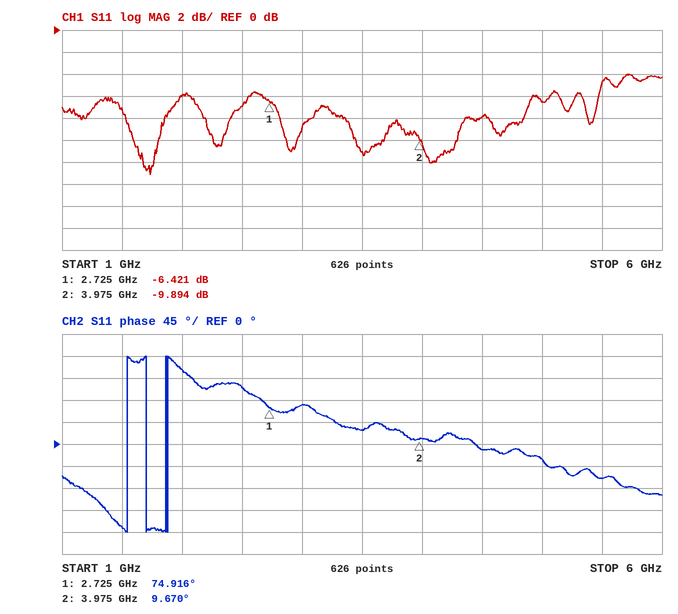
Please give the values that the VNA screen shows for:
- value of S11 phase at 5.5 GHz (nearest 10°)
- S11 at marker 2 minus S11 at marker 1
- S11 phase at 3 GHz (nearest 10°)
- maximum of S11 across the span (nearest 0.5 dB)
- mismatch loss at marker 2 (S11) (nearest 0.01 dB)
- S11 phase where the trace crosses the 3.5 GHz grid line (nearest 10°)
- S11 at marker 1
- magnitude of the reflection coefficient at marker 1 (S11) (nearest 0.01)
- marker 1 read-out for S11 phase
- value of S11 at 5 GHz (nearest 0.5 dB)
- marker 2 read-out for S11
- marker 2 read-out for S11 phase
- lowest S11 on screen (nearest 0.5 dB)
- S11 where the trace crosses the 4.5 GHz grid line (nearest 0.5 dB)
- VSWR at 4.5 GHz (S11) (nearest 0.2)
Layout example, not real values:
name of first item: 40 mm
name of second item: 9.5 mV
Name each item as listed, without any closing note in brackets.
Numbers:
value of S11 phase at 5.5 GHz: -70°
S11 at marker 2 minus S11 at marker 1: -3.473 dB
S11 phase at 3 GHz: 80°
maximum of S11 across the span: -4.0 dB
mismatch loss at marker 2 (S11): 0.47 dB
S11 phase where the trace crosses the 3.5 GHz grid line: 30°
S11 at marker 1: -6.421 dB
magnitude of the reflection coefficient at marker 1 (S11): 0.48
marker 1 read-out for S11 phase: 74.916°
value of S11 at 5 GHz: -6.5 dB
marker 2 read-out for S11: -9.894 dB
marker 2 read-out for S11 phase: 9.670°
lowest S11 on screen: -13.0 dB
S11 where the trace crosses the 4.5 GHz grid line: -8.0 dB
VSWR at 4.5 GHz (S11): 2.4
